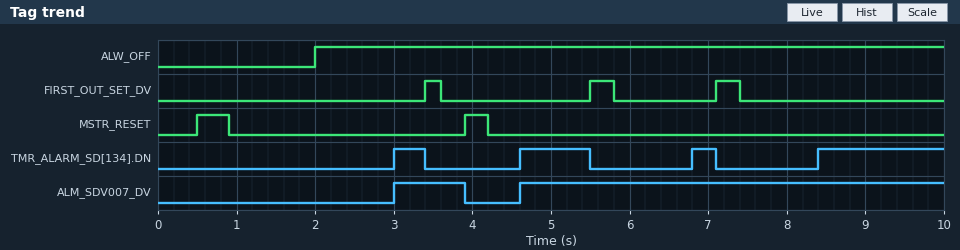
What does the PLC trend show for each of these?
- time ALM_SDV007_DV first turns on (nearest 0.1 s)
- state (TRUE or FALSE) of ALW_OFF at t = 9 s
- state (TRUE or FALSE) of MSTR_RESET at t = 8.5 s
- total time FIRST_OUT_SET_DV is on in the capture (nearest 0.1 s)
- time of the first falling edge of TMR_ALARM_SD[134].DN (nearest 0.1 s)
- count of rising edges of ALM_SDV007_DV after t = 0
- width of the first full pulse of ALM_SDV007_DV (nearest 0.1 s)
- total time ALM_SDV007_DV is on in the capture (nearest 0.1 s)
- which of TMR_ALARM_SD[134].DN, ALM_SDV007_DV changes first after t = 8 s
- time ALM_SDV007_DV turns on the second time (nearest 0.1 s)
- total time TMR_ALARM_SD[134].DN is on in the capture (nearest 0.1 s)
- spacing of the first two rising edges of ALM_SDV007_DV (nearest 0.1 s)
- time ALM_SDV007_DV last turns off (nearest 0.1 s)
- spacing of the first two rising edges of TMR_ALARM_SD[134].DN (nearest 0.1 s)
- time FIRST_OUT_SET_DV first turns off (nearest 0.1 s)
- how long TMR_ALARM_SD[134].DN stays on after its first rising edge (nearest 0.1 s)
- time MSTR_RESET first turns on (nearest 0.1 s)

3.0 s
TRUE
FALSE
0.8 s
3.4 s
2
0.9 s
6.3 s
TMR_ALARM_SD[134].DN
4.6 s
3.2 s
1.6 s
3.9 s
1.6 s
3.6 s
0.4 s
0.5 s
